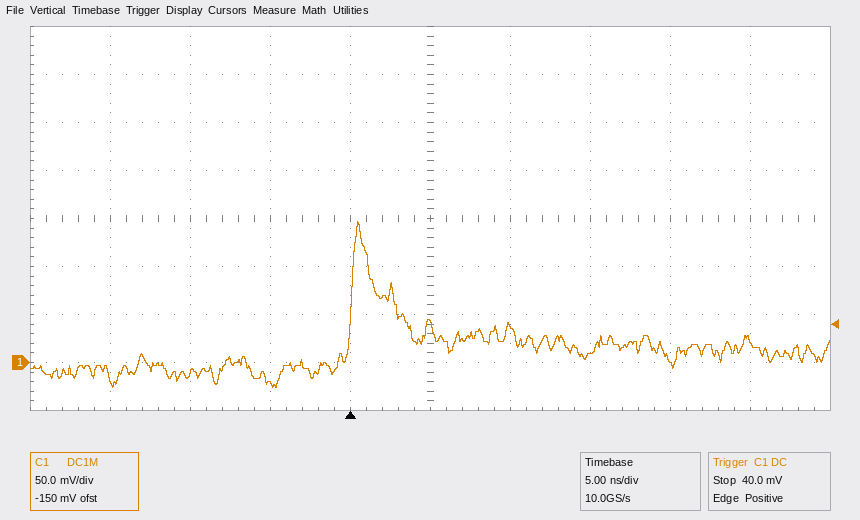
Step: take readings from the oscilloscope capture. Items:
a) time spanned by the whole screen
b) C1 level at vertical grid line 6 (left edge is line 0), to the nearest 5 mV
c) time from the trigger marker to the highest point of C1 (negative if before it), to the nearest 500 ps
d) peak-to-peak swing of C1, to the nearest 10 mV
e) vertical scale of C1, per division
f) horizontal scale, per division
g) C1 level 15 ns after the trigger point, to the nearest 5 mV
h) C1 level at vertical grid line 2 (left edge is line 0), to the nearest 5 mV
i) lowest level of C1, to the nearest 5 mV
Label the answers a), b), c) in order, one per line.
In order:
a) 50 ns
b) 35 mV
c) +500 ps
d) 170 mV
e) 50 mV
f) 5 ns
g) 10 mV
h) -10 mV
i) -25 mV
